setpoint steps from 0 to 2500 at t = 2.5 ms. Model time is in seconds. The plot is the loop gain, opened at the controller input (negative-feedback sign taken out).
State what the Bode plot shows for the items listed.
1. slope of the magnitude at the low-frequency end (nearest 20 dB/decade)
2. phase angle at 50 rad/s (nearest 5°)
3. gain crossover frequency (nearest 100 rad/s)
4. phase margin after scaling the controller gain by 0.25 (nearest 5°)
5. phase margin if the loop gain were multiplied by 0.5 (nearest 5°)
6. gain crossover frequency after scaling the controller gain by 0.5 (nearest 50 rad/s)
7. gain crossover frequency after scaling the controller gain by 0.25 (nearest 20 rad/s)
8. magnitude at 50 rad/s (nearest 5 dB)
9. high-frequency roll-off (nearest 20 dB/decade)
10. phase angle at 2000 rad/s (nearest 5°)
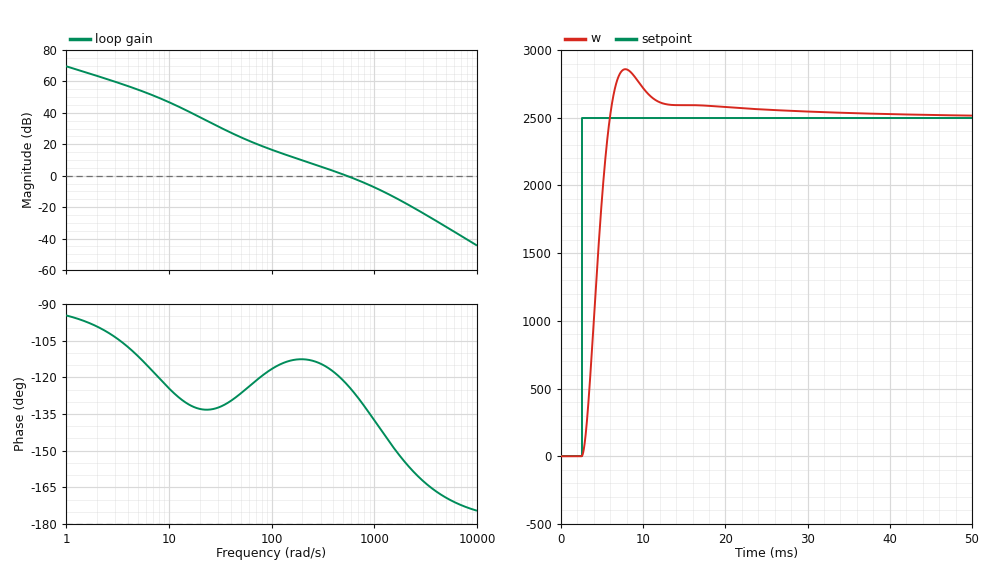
-20 dB/decade
-125°
500 rad/s
65°
65°
300 rad/s
160 rad/s
25 dB
-40 dB/decade
-155°
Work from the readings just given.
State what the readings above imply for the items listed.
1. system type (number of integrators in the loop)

1
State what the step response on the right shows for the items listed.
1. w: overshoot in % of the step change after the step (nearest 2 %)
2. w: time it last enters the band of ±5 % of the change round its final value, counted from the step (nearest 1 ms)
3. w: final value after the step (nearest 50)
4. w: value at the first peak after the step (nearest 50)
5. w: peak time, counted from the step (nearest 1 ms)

14 %
9 ms
2500
2850
5 ms
